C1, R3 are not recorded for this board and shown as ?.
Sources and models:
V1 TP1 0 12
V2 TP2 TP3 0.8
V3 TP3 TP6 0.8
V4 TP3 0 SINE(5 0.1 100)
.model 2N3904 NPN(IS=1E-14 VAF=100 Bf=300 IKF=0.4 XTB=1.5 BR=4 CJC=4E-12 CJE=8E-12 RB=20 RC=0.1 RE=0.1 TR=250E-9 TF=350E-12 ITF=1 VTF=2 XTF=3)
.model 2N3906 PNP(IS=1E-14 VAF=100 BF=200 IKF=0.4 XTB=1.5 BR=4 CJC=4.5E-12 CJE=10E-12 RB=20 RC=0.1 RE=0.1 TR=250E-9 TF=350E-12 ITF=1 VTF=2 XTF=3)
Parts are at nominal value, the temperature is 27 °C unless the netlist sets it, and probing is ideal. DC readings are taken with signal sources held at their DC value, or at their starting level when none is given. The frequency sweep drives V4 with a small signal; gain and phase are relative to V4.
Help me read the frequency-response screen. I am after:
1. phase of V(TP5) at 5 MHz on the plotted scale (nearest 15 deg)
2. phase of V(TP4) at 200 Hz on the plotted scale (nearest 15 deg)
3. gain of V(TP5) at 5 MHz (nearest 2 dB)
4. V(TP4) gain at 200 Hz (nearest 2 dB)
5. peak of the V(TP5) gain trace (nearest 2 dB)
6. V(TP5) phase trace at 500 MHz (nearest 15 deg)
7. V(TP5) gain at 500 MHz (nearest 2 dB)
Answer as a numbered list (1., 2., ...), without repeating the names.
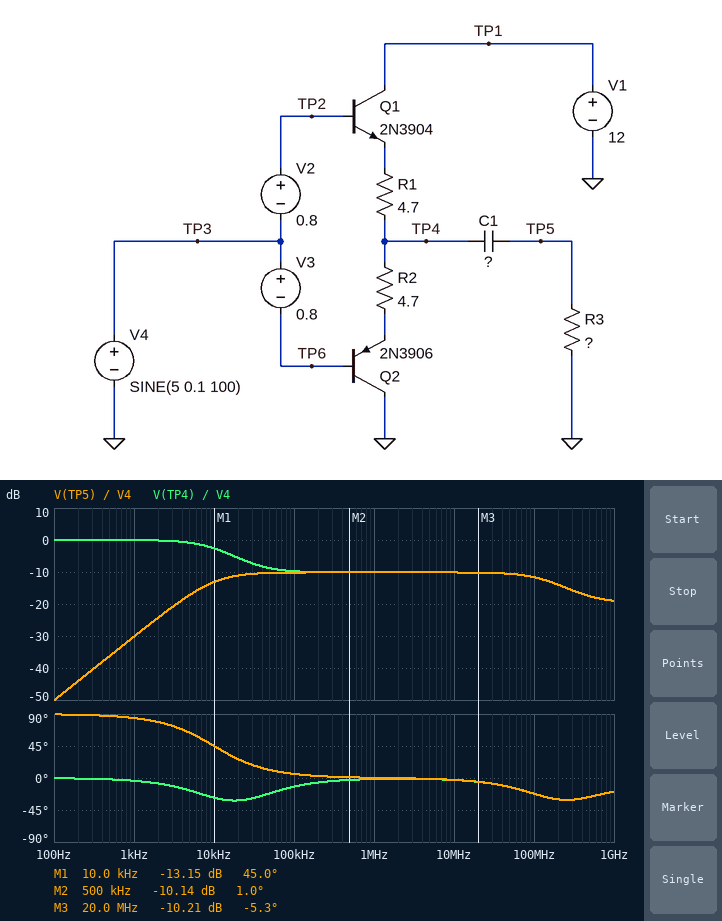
1. 0 deg
2. 0 deg
3. -10 dB
4. 0 dB
5. -10 dB
6. -30 deg
7. -18 dB
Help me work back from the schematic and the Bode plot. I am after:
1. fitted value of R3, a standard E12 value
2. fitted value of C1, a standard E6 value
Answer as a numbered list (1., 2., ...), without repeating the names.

1. 1.5 Ω
2. 3.3 µF
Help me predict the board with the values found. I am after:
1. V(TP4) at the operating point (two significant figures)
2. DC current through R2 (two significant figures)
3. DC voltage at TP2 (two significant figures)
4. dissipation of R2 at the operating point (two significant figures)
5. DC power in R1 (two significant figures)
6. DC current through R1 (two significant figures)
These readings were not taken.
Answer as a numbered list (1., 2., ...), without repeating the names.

1. 5.0 V
2. 15 mA
3. 5.8 V
4. 1.1 mW
5. 1.1 mW
6. 15 mA
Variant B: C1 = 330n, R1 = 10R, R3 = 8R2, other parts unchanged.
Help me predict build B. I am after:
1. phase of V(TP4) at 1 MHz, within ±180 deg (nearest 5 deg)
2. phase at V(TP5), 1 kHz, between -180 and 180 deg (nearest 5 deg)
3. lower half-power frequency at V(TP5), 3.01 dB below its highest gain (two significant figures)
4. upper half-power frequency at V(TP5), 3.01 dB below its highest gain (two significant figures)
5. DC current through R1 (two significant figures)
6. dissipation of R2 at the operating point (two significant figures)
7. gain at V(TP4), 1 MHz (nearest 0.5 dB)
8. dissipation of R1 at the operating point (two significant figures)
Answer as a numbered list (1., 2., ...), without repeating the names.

1. 0 deg
2. 90 deg
3. 38 kHz
4. 390 MHz
5. 11 mA
6. 580 µW
7. -4.0 dB
8. 1.2 mW
